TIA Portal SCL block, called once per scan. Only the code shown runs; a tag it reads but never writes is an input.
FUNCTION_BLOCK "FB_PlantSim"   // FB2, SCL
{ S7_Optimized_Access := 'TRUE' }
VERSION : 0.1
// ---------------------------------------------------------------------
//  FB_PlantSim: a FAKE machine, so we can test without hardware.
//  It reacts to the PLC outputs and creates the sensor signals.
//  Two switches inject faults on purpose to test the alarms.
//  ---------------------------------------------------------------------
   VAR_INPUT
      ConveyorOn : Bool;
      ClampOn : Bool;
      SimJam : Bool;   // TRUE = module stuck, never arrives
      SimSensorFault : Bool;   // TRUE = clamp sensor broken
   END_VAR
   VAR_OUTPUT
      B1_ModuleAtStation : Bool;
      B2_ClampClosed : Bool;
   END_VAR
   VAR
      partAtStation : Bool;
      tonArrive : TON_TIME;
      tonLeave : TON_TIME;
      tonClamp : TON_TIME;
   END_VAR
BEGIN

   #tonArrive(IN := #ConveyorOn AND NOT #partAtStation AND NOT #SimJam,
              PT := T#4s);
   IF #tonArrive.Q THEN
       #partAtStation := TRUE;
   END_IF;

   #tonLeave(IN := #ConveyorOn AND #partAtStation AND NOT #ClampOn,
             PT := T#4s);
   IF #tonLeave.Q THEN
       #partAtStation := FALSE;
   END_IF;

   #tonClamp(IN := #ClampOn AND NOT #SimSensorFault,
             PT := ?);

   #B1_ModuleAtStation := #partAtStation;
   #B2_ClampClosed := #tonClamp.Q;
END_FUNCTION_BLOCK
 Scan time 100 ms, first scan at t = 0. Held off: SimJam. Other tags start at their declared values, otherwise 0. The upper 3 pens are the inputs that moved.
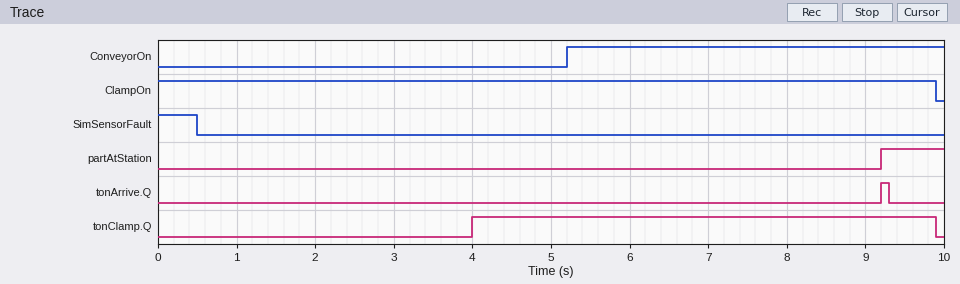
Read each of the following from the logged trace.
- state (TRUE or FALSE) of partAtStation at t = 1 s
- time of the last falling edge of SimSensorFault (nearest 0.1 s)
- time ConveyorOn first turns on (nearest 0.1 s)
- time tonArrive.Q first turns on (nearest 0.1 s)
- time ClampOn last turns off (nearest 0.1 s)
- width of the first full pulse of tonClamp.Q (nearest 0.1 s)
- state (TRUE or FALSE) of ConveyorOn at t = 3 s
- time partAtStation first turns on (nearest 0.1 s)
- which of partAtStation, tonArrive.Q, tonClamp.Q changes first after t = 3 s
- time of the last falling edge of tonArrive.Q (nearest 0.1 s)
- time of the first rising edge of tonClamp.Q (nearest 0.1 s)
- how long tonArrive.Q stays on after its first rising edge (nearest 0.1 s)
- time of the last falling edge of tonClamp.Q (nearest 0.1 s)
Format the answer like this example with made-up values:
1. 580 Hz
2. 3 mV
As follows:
1. FALSE
2. 0.5 s
3. 5.2 s
4. 9.2 s
5. 9.9 s
6. 5.9 s
7. FALSE
8. 9.2 s
9. tonClamp.Q
10. 9.3 s
11. 4.0 s
12. 0.1 s
13. 9.9 s
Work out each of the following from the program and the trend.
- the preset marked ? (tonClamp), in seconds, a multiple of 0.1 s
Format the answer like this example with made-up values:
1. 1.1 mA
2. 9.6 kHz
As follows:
1. 3.5 s
